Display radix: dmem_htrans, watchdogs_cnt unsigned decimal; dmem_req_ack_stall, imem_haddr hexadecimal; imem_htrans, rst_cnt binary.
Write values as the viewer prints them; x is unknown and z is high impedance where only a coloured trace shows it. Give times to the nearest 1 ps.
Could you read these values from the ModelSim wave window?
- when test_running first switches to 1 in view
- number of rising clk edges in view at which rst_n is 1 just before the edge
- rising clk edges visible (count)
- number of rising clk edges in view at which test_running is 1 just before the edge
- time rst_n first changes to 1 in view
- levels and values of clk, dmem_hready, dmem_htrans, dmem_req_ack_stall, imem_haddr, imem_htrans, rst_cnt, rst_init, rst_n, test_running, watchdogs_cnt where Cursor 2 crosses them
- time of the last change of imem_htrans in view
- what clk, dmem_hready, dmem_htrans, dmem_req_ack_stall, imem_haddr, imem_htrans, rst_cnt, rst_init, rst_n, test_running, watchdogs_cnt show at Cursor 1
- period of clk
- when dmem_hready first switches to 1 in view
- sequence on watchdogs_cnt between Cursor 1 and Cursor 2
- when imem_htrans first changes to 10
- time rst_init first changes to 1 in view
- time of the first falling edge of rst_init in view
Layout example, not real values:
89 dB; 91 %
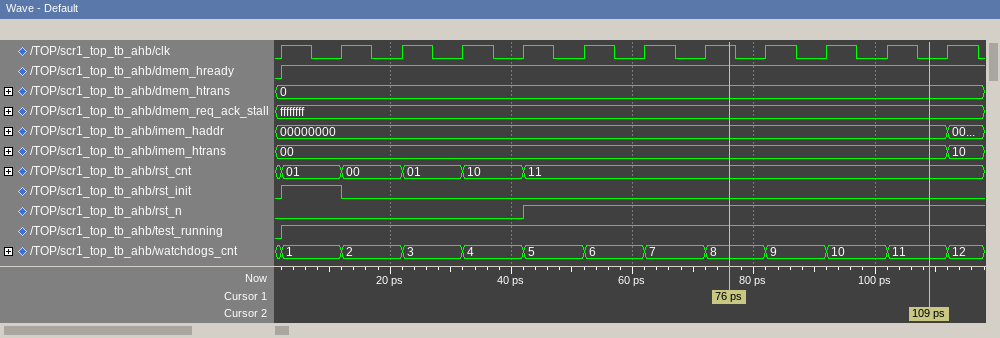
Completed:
2 ps; 7; 12; 11; 42 ps; clk=0, dmem_hready=1, dmem_htrans=0, dmem_req_ack_stall=ffffffff, imem_haddr=00000000, imem_htrans=00, rst_cnt=11, rst_init=0, rst_n=1, test_running=1, watchdogs_cnt=11; 112 ps; clk=1, dmem_hready=1, dmem_htrans=0, dmem_req_ack_stall=ffffffff, imem_haddr=00000000, imem_htrans=00, rst_cnt=11, rst_init=0, rst_n=1, test_running=1, watchdogs_cnt=8; 10 ps; 2 ps; 8, 9, 10, 11; 112 ps; 2 ps; 12 ps
